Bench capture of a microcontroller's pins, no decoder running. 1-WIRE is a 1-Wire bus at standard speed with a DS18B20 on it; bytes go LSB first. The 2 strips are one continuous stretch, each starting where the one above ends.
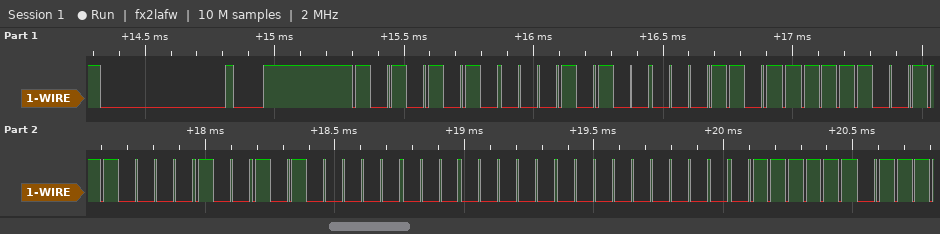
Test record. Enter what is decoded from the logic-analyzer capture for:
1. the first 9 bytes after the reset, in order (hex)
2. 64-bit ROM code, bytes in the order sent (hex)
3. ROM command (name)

55 28 D8 CF 21 05 00 00 FC
28 D8 CF 21 05 00 00 FC
Match ROM
